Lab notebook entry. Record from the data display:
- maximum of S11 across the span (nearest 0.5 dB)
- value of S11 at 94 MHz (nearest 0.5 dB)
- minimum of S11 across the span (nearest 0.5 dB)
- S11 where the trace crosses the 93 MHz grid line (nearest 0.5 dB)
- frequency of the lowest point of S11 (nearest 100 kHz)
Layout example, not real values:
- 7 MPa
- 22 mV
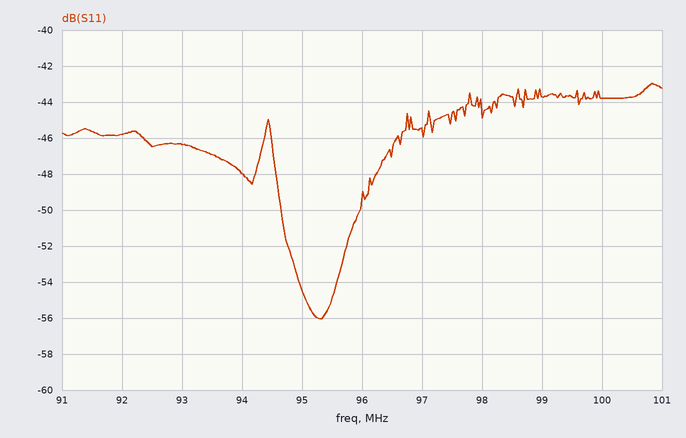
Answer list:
- -43.0 dB
- -48.0 dB
- -56.0 dB
- -46.5 dB
- 95.3 MHz
